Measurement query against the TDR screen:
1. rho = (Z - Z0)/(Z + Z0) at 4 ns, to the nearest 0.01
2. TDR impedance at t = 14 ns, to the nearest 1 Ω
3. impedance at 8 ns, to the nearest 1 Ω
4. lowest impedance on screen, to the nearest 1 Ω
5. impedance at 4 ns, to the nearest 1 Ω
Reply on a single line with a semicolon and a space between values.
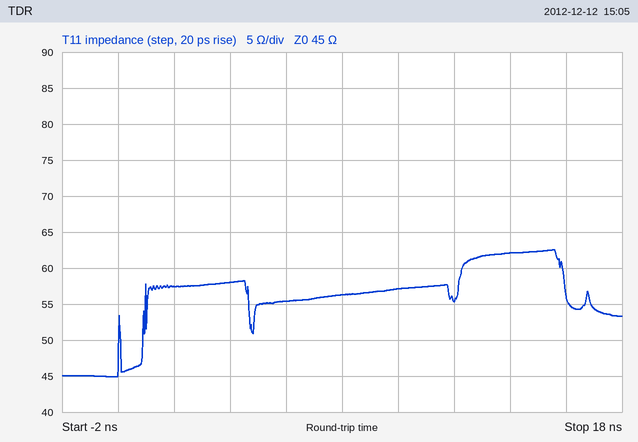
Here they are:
+0.13; 62 Ω; 56 Ω; 45 Ω; 58 Ω
